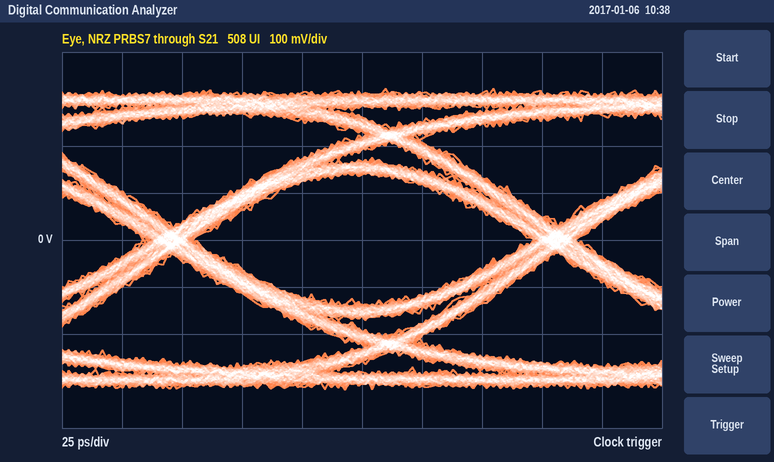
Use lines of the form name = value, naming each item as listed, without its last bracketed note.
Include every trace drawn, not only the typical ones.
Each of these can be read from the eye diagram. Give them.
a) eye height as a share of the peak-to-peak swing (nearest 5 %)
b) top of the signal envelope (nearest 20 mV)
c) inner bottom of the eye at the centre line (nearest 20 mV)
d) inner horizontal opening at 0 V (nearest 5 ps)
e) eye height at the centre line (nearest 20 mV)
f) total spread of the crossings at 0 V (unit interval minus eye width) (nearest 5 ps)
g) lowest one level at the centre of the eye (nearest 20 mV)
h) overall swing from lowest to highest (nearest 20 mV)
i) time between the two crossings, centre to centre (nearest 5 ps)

eye height as a share of the peak-to-peak swing = 45 %
top of the signal envelope = 320 mV
inner bottom of the eye at the centre line = -140 mV
inner horizontal opening at 0 V = 140 ps
eye height at the centre line = 280 mV
total spread of the crossings at 0 V (unit interval minus eye width) = 20 ps
lowest one level at the centre of the eye = 140 mV
overall swing from lowest to highest = 640 mV
time between the two crossings, centre to centre = 160 ps
